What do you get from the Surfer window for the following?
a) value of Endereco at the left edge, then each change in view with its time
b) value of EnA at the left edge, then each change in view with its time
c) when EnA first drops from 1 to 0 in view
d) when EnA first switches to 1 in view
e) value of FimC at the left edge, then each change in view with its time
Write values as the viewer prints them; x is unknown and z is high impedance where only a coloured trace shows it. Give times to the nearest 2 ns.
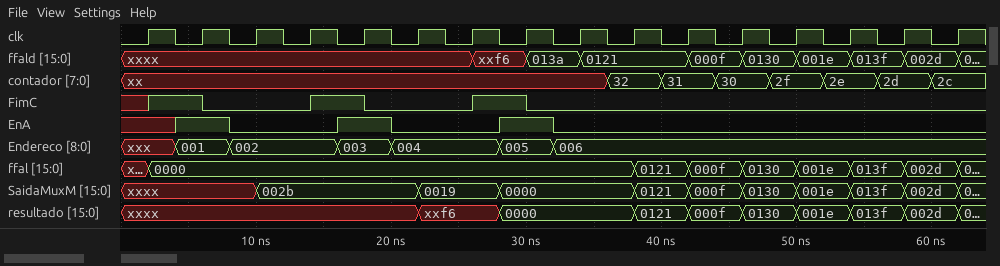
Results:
xxx, 001 at 4 ns, 002 at 8 ns, 003 at 16 ns, 004 at 20 ns, 005 at 28 ns, 006 at 32 ns
x, 1 at 4 ns, 0 at 8 ns, 1 at 16 ns, 0 at 20 ns, 1 at 28 ns, 0 at 32 ns
8 ns
4 ns
x, 1 at 2 ns, 0 at 6 ns, 1 at 14 ns, 0 at 18 ns, 1 at 26 ns, 0 at 30 ns
